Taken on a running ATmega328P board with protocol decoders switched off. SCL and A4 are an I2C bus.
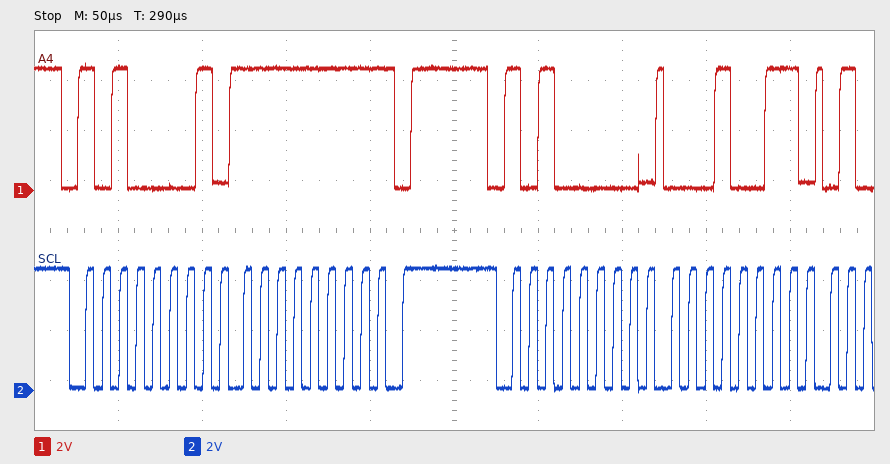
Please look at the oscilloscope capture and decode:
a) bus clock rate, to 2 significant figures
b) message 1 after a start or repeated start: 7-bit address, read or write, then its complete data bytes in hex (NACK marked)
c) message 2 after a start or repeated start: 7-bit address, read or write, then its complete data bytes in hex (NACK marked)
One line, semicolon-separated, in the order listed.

100 kHz; 0x50 read: FF NACK; 0x50 write: 13
